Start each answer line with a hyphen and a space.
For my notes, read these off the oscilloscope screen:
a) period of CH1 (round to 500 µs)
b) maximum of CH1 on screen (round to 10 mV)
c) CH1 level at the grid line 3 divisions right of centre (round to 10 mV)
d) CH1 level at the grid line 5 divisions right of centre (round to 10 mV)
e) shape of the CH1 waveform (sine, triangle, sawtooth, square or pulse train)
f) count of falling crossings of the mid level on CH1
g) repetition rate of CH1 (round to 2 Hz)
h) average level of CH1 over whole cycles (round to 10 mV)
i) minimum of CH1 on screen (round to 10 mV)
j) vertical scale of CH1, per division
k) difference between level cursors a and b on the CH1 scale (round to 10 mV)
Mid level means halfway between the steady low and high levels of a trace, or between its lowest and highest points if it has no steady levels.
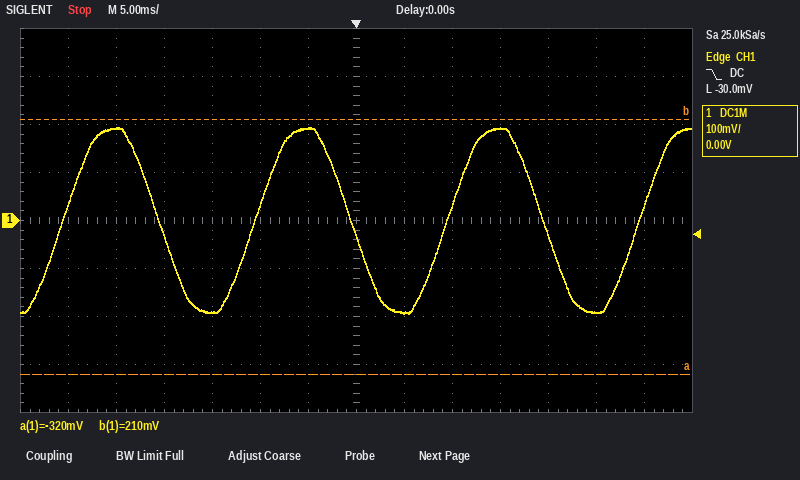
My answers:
- 20.0 ms
- 190 mV
- 190 mV
- -190 mV
- sine
- 3
- 50 Hz
- 0 mV
- -190 mV
- 100 mV
- 530 mV
